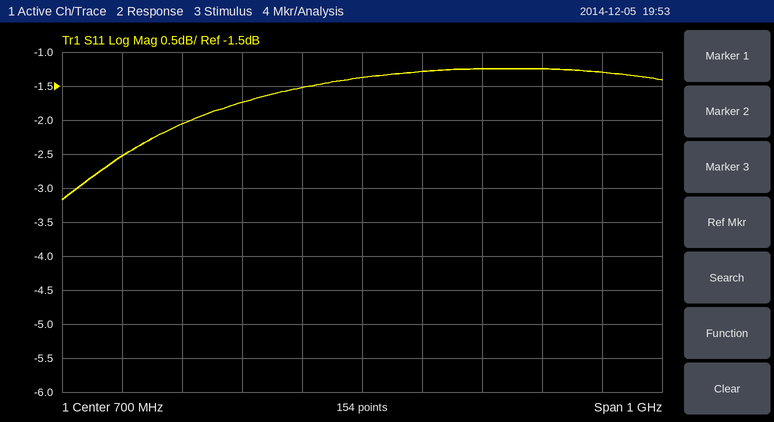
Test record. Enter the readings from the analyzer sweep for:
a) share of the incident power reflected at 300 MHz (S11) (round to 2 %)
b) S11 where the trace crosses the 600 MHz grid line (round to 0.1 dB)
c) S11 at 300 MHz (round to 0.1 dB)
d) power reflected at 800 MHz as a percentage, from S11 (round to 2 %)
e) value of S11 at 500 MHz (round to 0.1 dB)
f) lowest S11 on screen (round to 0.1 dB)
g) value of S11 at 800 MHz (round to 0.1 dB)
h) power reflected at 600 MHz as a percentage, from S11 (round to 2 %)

56 %
-1.5 dB
-2.5 dB
74 %
-1.7 dB
-3.2 dB
-1.3 dB
70 %
